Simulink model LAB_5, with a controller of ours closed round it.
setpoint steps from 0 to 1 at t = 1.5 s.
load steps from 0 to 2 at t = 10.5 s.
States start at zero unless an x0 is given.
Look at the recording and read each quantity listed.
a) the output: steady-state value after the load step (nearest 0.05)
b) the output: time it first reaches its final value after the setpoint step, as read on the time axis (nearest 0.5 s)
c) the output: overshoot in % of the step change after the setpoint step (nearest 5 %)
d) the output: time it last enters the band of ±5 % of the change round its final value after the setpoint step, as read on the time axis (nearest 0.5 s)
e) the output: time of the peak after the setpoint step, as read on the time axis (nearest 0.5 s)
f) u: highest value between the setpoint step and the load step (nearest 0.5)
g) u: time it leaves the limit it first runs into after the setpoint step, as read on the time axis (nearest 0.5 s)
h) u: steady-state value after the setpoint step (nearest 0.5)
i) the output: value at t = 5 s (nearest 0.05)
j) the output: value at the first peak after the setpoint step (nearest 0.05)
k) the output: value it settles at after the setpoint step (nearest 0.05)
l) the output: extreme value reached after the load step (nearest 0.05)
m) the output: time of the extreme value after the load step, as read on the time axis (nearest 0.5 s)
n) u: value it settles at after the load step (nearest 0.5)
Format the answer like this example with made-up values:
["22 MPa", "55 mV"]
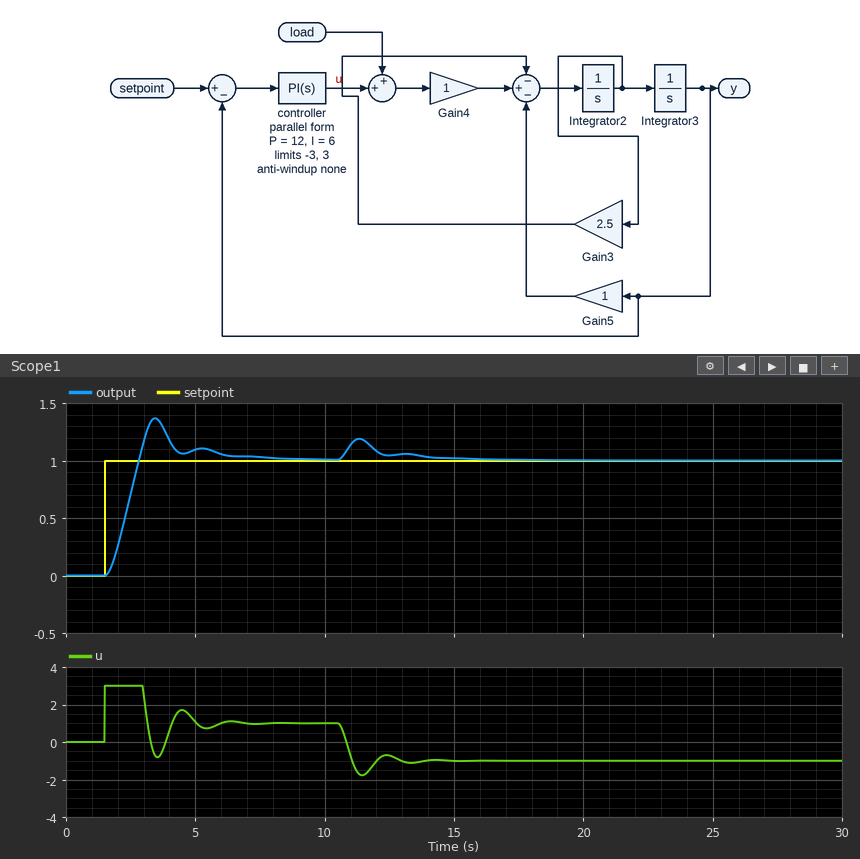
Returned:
["1.00", "3.0 s", "35 %", "6.0 s", "3.5 s", "3.0", "3.0 s", "1.0", "1.10", "1.35", "1.00", "1.20", "11.5 s", "-1.0"]
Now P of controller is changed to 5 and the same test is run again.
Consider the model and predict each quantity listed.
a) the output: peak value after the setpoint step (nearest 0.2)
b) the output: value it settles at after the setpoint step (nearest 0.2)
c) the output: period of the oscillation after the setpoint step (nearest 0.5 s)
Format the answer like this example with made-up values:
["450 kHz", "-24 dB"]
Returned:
["1.6", "1.0", "3.0 s"]
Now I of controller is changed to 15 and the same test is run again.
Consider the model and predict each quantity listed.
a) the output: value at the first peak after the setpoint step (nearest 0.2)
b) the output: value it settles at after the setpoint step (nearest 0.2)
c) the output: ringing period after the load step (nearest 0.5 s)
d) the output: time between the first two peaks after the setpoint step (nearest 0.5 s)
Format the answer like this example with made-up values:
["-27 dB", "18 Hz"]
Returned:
["1.6", "1.0", "2.0 s", "2.0 s"]
